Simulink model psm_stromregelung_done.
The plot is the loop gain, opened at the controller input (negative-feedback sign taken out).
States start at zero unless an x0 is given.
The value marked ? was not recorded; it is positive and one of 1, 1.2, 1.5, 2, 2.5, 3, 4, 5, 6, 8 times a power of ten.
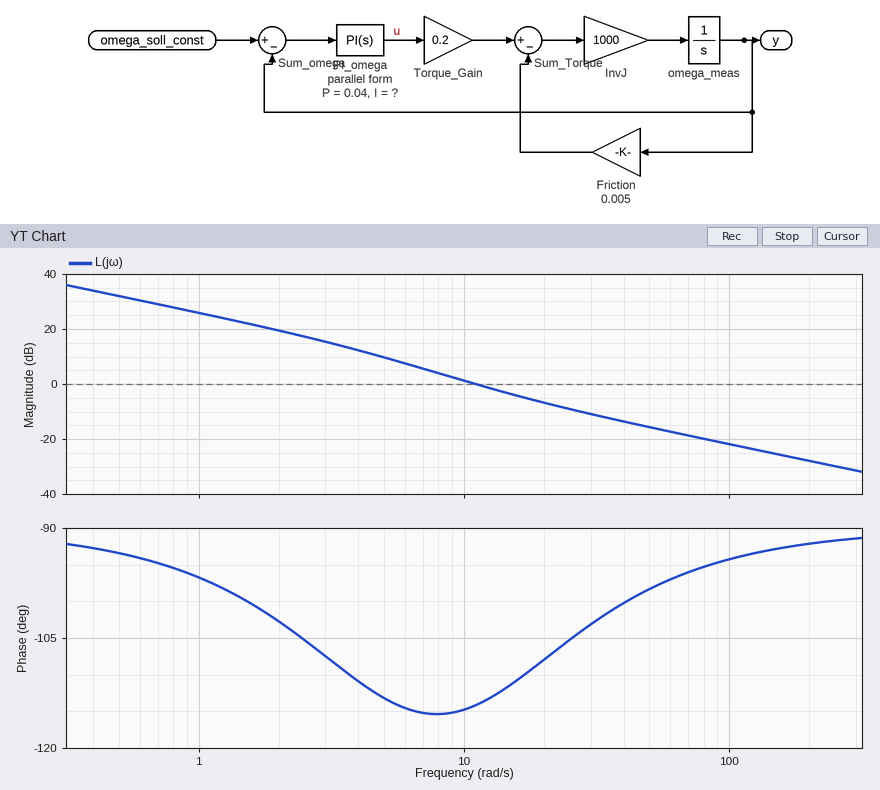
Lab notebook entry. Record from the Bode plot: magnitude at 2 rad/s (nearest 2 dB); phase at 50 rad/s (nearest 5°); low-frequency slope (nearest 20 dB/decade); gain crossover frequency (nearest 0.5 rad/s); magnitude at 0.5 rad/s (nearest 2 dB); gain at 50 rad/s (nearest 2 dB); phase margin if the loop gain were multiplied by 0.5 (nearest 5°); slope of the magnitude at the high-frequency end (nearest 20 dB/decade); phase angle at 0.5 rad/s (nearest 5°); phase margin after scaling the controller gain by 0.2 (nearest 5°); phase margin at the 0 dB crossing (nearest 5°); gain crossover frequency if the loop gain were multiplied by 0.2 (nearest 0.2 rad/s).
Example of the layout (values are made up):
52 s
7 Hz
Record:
20 dB
-100°
-20 dB/decade
11.0 rad/s
32 dB
-16 dB
65°
-20 dB/decade
-95°
70°
65°
3.4 rad/s
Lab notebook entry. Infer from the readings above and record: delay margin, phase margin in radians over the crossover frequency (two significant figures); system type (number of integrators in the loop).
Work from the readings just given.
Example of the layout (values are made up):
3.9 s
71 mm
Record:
0.10 s
1
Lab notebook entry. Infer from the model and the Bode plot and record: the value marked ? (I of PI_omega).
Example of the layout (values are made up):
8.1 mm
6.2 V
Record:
0.5
